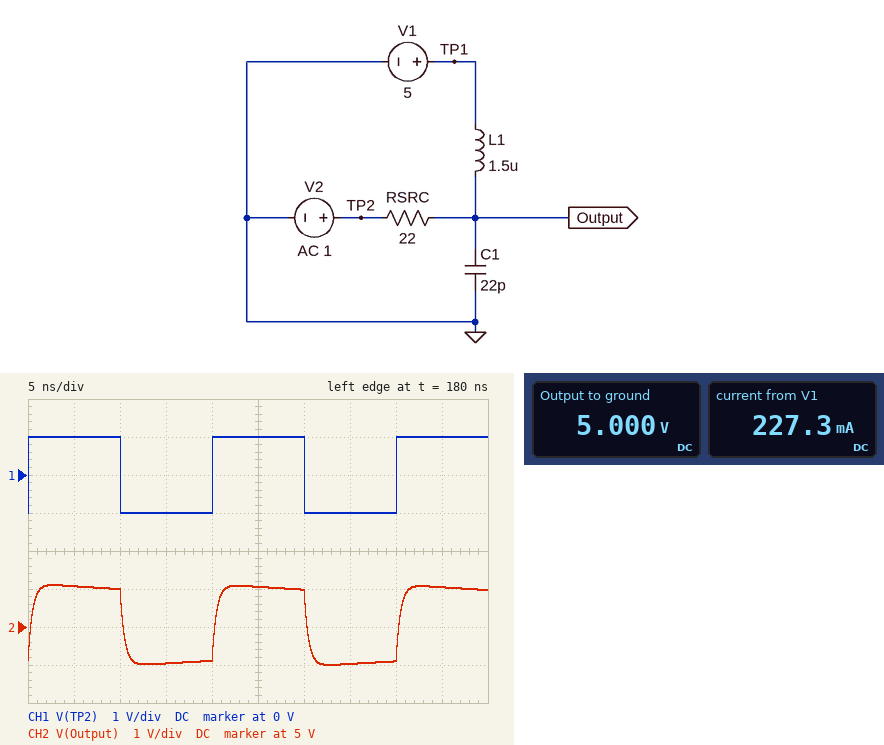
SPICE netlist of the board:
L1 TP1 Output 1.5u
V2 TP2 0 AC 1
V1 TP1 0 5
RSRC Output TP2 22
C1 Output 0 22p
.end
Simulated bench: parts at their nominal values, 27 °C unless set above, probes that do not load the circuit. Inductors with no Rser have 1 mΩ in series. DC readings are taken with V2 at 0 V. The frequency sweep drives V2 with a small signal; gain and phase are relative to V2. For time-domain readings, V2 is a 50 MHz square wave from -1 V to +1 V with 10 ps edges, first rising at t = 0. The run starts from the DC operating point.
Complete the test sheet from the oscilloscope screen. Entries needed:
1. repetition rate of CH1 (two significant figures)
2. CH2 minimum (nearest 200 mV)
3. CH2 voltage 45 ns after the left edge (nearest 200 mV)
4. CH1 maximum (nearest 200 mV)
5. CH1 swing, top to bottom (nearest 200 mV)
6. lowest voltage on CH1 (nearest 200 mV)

50 MHz
4.0 V
6.0 V
1.0 V
2.0 V
-1.0 V
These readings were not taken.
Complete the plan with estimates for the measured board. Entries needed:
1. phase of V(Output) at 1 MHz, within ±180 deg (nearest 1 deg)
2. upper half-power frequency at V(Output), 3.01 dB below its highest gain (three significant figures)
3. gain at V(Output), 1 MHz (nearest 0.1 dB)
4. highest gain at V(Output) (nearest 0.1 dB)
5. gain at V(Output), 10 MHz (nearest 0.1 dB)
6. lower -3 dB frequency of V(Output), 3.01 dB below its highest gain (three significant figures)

67 deg
331 MHz
-8.1 dB
0 dB
-0.2 dB
2.32 MHz
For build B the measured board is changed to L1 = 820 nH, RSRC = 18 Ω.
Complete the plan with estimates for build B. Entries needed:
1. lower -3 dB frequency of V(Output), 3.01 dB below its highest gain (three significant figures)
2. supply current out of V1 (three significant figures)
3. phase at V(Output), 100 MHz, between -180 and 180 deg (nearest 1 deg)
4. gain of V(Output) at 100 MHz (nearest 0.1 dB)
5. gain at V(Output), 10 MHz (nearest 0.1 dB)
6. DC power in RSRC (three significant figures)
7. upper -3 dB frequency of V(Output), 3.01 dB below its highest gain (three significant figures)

3.46 MHz
278 mA
-12 deg
-0.2 dB
-0.4 dB
1.39 W
405 MHz
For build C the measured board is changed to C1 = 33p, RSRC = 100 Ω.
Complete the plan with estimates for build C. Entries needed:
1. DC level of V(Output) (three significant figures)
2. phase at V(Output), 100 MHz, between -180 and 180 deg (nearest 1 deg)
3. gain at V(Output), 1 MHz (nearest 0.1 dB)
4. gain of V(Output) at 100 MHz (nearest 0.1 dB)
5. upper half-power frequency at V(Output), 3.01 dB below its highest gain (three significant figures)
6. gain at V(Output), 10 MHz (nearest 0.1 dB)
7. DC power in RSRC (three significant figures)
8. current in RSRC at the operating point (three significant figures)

5.00 V
-63 deg
-20.5 dB
-6.9 dB
57.2 MHz
-2.4 dB
250 mW
50.0 mA
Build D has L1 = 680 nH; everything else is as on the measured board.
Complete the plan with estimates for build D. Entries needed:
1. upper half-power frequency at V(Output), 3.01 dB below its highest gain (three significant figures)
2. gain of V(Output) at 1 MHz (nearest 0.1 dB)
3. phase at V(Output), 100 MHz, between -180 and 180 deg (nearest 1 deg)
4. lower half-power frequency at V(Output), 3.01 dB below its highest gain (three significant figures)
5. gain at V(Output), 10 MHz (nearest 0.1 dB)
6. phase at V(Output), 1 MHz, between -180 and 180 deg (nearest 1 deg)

334 MHz
-14.4 dB
-14 deg
5.07 MHz
-0.9 dB
79 deg
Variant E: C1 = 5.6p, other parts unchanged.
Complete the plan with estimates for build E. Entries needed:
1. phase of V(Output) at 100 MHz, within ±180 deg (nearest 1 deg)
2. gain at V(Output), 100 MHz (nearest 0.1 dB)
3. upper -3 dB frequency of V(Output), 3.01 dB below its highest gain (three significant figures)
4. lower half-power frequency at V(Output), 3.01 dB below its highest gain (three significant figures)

-3 deg
0 dB
1.29 GHz
2.33 MHz
